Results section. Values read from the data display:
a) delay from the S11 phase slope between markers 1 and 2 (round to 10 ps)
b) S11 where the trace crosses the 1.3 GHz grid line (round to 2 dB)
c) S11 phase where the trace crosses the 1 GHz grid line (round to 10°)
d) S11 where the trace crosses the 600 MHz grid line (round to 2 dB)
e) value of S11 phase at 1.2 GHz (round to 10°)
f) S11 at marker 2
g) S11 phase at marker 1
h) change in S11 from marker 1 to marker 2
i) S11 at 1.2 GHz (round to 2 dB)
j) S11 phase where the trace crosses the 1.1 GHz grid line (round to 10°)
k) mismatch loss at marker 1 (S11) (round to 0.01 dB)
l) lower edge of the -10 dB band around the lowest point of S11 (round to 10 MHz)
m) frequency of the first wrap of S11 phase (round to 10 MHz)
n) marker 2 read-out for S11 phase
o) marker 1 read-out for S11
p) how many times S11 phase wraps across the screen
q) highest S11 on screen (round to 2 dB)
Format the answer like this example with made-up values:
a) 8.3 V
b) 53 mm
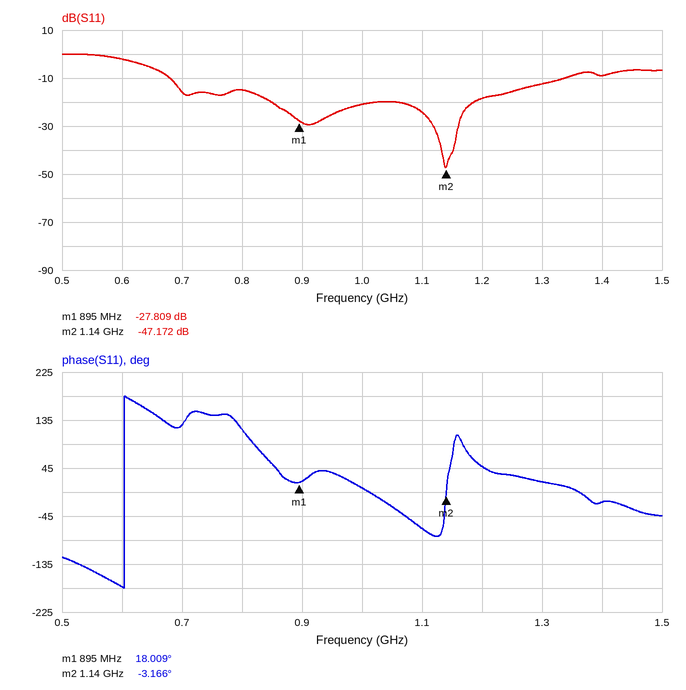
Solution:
a) 240 ps
b) -12 dB
c) 10°
d) -2 dB
e) 50°
f) -47.172 dB
g) 18.009°
h) -19.363 dB
i) -18 dB
j) -70°
k) 0.01 dB
l) 680 MHz
m) 600 MHz
n) -3.166°
o) -27.809 dB
p) 1
q) 0 dB
